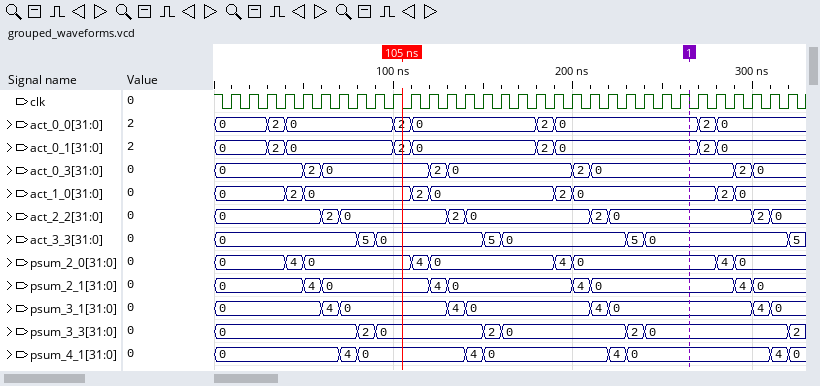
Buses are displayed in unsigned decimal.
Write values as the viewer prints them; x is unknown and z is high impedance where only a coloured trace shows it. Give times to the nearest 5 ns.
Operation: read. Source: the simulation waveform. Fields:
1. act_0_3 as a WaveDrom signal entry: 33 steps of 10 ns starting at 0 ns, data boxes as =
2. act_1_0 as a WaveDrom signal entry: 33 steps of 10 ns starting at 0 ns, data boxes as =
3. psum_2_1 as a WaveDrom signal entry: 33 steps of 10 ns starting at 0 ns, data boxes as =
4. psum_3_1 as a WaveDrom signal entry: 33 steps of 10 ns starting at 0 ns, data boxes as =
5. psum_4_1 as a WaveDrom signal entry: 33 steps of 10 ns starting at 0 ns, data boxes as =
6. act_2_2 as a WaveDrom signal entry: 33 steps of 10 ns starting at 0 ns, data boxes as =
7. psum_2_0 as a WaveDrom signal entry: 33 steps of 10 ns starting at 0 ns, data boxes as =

{name: 'act_0_3', wave: '=....==.....==......==.......==..', data: '0 2 0 2 0 2 0 2 0'}
{name: 'act_1_0', wave: '=...==.....==......==.......==...', data: '0 2 0 2 0 2 0 2 0'}
{name: 'psum_2_1', wave: '=....==.....==......==.......==..', data: '0 4 0 4 0 4 0 4 0'}
{name: 'psum_3_1', wave: '=.....==.....==......==.......==.', data: '0 4 0 4 0 4 0 4 0'}
{name: 'psum_4_1', wave: '=......==.....==......==.......==', data: '0 4 0 4 0 4 0 4 0'}
{name: 'act_2_2', wave: '=.....==.....==......==.......==.', data: '0 2 0 2 0 2 0 2 0'}
{name: 'psum_2_0', wave: '=...==.....==......==.......==...', data: '0 4 0 4 0 4 0 4 0'}
